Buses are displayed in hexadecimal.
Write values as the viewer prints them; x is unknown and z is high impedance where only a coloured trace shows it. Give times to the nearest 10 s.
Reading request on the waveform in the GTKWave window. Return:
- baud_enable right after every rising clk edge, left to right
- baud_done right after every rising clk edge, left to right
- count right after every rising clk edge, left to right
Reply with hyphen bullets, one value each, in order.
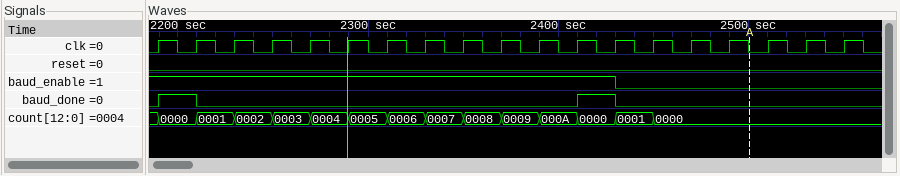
- 1 1 1 1 1 1 1 1 1 1 1 1 0 0 0 0 0 0 0
- 1 0 0 0 0 0 0 0 0 0 0 1 0 0 0 0 0 0 0
- 0000, 0001, 0002, 0003, 0004, 0005, 0006, 0007, 0008, 0009, 000A, 0000, 0001, 0000, 0000, 0000, 0000, 0000, 0000
